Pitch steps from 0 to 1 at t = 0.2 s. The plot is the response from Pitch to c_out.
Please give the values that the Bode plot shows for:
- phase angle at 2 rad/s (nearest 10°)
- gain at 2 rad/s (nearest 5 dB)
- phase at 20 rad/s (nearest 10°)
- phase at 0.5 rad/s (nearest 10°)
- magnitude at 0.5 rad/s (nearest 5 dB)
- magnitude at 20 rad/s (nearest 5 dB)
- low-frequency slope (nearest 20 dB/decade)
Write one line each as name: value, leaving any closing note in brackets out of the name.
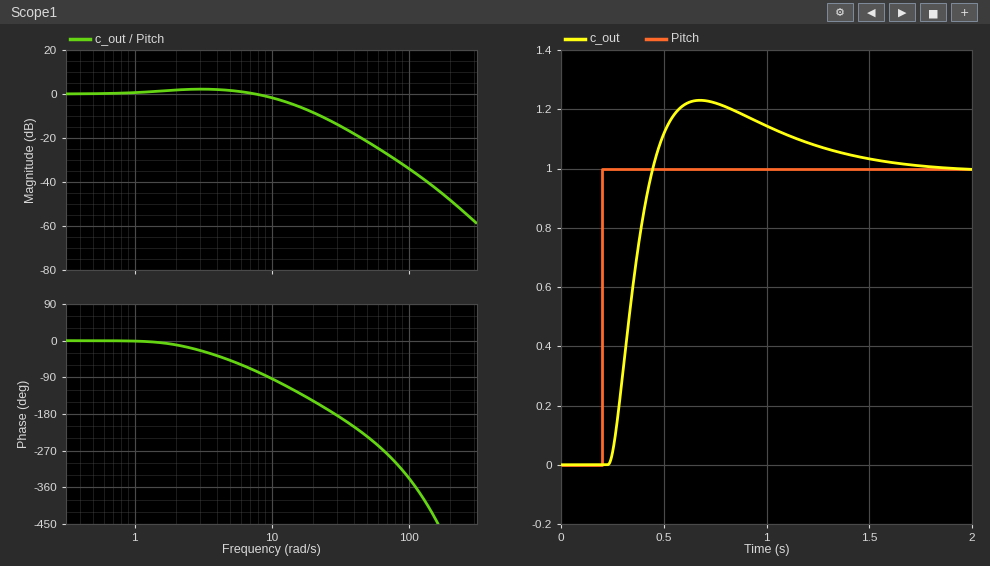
phase angle at 2 rad/s: -10°
gain at 2 rad/s: 0 dB
phase at 20 rad/s: -150°
phase at 0.5 rad/s: 0°
magnitude at 0.5 rad/s: 0 dB
magnitude at 20 rad/s: -10 dB
low-frequency slope: 0 dB/decade
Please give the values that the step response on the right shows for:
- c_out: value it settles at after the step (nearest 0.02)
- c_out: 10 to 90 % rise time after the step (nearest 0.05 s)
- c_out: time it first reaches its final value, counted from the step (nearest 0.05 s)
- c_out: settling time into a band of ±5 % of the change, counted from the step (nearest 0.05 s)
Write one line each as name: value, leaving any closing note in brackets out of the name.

c_out: value it settles at after the step: 1.00
c_out: 10 to 90 % rise time after the step: 0.15 s
c_out: time it first reaches its final value, counted from the step: 0.25 s
c_out: settling time into a band of ±5 % of the change, counted from the step: 1.20 s
